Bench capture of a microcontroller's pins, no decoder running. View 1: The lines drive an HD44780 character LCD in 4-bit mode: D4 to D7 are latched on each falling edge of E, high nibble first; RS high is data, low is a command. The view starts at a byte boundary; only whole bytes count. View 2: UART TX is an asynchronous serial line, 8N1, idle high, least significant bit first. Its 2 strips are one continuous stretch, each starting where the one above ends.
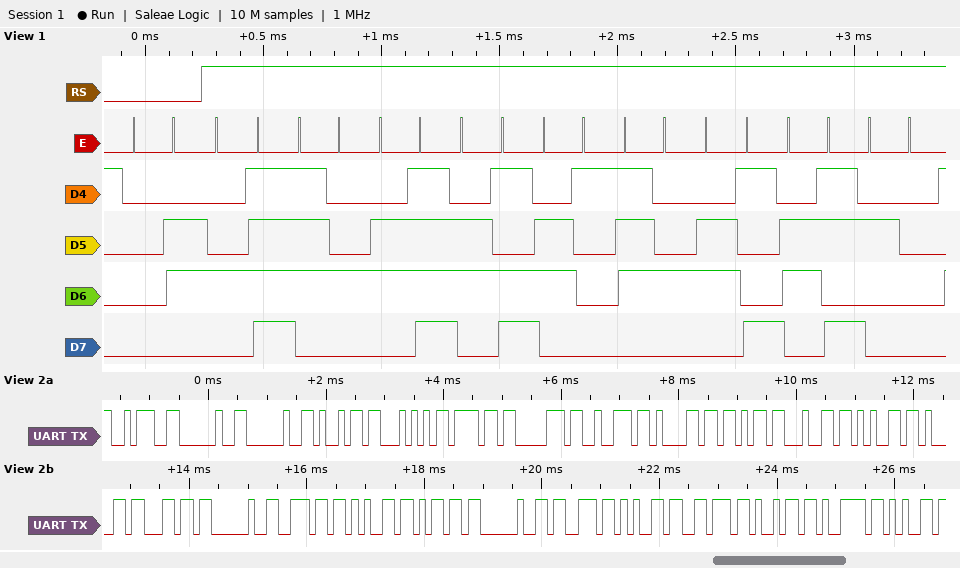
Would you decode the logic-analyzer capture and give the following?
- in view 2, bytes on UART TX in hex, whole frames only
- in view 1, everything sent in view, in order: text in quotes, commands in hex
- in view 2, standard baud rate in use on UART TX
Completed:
0x3A 0x20 0x20 0x69 0x54 0x6F 0x70 0x72 0x61 0x6B 0x64 0x65 0x61 0x6C 0x20 0x6E 0x65 0x6D 0x20 0x73 0x65 0x76 0x69 0x79 0x65
0x06 "Otomatik "
9600 baud
